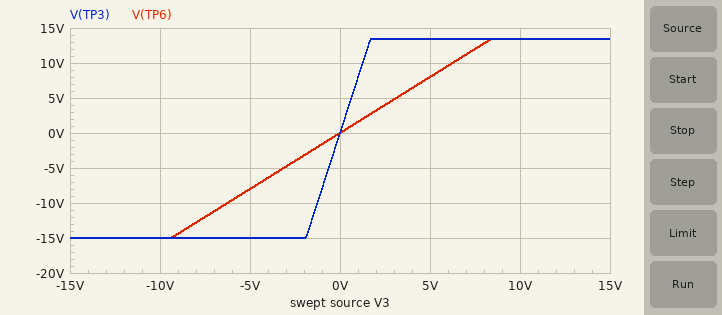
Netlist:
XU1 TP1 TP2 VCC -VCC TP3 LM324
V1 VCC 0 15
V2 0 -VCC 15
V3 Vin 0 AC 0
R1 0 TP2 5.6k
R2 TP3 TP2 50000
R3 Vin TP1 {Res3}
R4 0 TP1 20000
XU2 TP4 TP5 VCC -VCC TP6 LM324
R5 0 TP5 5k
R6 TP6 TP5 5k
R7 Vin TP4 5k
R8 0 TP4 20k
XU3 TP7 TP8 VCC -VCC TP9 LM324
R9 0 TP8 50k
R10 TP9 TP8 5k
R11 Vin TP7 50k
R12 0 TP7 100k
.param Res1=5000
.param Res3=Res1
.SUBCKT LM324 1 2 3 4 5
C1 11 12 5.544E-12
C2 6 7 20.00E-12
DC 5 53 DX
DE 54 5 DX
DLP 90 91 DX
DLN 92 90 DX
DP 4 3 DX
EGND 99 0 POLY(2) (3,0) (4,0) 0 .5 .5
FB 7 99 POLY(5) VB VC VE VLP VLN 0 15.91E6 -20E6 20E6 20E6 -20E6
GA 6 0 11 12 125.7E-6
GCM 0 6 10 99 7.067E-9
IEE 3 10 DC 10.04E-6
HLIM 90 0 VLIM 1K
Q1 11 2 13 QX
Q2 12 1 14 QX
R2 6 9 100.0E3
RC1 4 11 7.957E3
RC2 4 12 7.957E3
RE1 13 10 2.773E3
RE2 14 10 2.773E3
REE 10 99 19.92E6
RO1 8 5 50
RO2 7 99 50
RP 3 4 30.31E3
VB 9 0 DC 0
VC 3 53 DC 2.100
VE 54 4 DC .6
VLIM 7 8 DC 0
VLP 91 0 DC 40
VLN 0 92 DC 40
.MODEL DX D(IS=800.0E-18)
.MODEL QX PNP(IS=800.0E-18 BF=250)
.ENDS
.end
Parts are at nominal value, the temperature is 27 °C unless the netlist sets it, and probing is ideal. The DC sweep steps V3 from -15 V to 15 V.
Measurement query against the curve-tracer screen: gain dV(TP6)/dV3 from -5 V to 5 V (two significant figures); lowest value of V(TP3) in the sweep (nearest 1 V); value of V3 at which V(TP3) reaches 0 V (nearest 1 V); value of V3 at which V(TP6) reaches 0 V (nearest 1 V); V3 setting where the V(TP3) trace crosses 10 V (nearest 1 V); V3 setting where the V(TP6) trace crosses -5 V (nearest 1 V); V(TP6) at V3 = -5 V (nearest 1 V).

1.6 V/V
-15 V
0 V
0 V
1 V
-3 V
-8 V
